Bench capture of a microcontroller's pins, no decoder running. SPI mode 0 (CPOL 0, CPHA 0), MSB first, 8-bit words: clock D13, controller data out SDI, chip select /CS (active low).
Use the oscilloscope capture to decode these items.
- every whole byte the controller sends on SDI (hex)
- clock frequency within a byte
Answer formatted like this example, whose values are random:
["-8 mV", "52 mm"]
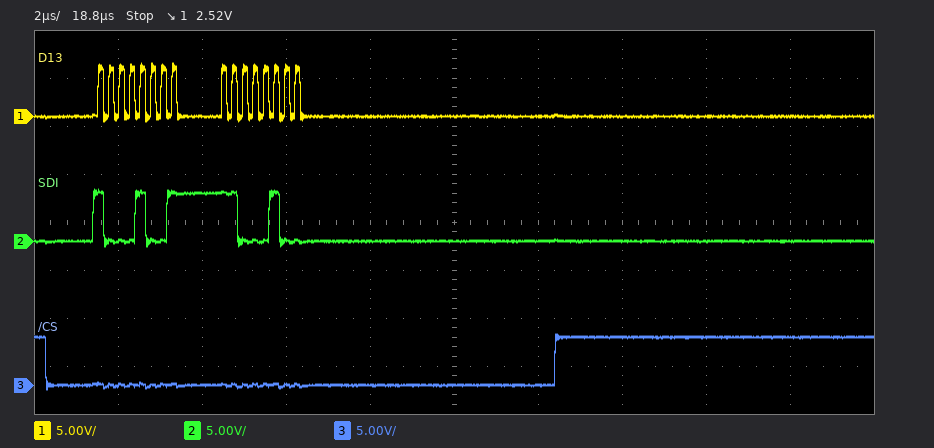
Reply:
["89 C4", "4 MHz"]
